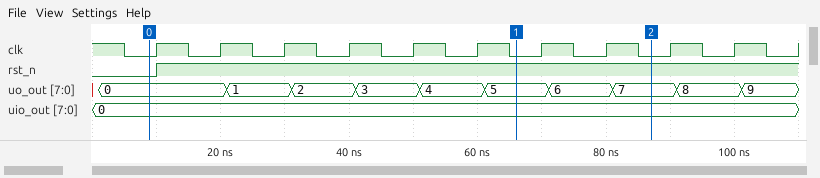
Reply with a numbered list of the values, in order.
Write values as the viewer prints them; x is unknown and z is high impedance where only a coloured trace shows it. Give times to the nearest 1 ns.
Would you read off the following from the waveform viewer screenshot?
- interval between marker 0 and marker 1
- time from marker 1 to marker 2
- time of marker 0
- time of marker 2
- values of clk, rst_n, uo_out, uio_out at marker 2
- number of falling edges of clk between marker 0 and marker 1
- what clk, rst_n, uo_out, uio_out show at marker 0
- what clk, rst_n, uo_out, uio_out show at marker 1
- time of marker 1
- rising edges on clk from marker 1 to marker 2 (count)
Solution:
1. 57 ns
2. 21 ns
3. 9 ns
4. 87 ns
5. clk=0, rst_n=1, uo_out=7, uio_out=0
6. 6
7. clk=0, rst_n=0, uo_out=0, uio_out=0
8. clk=0, rst_n=1, uo_out=5, uio_out=0
9. 66 ns
10. 2
